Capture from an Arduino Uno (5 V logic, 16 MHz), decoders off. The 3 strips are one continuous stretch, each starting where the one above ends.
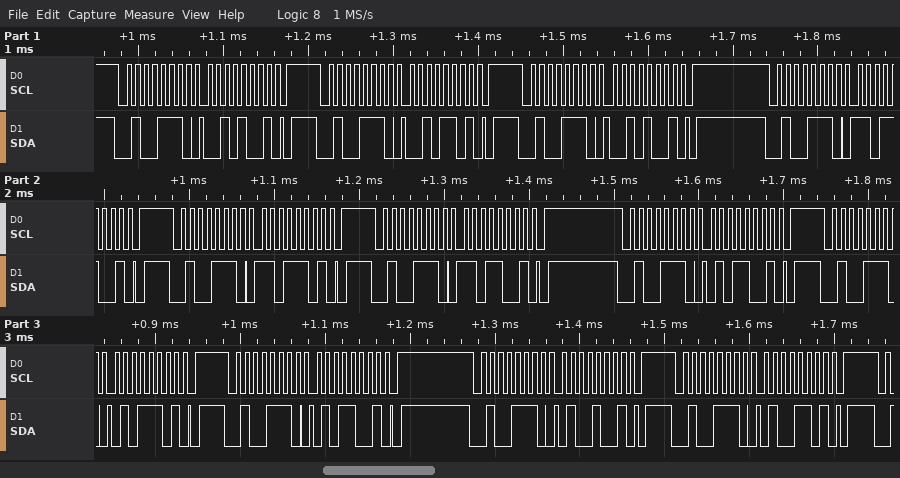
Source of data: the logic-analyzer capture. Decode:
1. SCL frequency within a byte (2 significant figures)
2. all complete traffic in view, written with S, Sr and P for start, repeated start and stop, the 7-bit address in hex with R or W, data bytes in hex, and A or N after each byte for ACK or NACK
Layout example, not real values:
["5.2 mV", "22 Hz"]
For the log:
["100 kHz", "S 27W A 29 A P S 27W A 2D A P S 27W A 29 A P S 27W A D9 A P S 27W A DD A P S 27W A D9 A P S 27W A 59 A P S 27W A 5D A P S 27W A 59 A P S 27W A 49 A P S 27W A 4D A P"]
